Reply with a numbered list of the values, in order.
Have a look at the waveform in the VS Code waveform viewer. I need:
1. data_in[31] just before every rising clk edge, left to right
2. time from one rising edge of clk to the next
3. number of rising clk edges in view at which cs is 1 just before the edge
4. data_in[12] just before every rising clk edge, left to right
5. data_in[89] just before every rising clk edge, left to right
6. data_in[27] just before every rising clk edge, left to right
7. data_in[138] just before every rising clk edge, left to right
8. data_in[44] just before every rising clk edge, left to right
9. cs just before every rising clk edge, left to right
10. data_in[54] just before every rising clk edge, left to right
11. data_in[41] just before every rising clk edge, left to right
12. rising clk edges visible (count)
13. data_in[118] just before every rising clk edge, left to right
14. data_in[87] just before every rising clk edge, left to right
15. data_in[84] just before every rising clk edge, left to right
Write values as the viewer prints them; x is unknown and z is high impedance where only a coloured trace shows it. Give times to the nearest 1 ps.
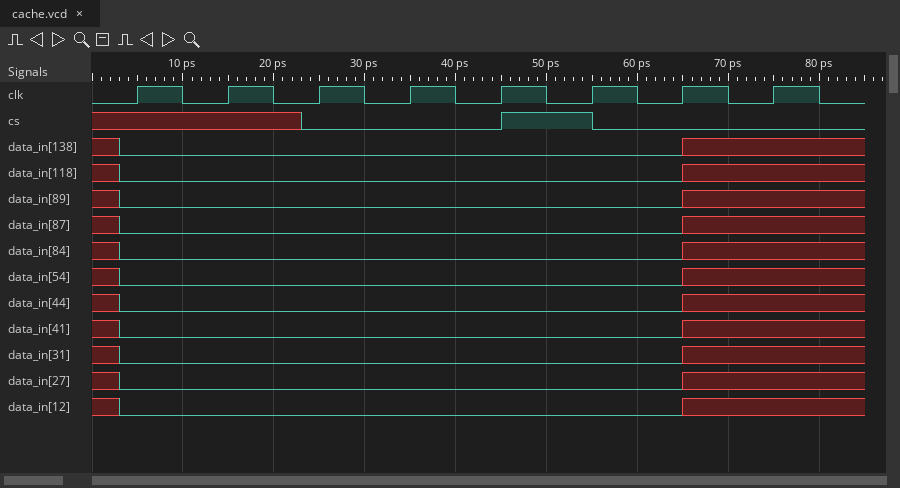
1. 0 0 0 0 0 0 0 x
2. 10 ps
3. 1
4. 0 0 0 0 0 0 0 x
5. 0 0 0 0 0 0 0 x
6. 0 0 0 0 0 0 0 x
7. 0 0 0 0 0 0 0 x
8. 0 0 0 0 0 0 0 x
9. x x 0 0 0 1 0 0
10. 0 0 0 0 0 0 0 x
11. 0 0 0 0 0 0 0 x
12. 8
13. 0 0 0 0 0 0 0 x
14. 0 0 0 0 0 0 0 x
15. 0 0 0 0 0 0 0 x
